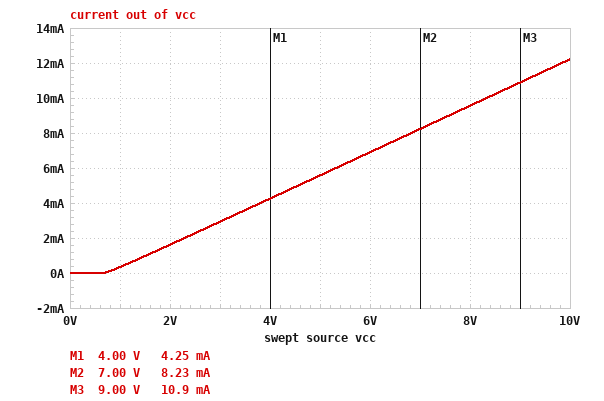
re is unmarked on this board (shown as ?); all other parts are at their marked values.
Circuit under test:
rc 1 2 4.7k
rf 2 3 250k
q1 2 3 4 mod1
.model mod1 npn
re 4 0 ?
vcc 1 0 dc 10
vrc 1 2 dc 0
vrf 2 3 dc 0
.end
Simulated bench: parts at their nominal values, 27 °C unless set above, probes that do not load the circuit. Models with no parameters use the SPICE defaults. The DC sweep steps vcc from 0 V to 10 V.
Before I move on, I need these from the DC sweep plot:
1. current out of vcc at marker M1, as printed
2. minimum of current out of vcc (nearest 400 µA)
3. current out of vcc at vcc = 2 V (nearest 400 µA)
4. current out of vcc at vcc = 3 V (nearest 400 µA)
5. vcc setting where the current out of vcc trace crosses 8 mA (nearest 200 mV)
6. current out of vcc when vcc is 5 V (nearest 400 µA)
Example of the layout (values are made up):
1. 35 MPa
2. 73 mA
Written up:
1. 4.25 mA
2. 0 A
3. 1.6 mA
4. 2.8 mA
5. 6.8 V
6. 5.6 mA
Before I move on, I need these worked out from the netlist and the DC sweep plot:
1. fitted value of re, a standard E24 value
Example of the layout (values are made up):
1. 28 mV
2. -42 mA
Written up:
1. 750 Ω
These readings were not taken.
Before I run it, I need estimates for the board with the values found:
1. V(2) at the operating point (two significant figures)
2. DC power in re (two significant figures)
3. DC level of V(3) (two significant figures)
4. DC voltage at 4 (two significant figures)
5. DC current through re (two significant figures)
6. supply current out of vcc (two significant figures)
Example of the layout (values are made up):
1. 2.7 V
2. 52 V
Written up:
1. 10 V
2. 110 mW
3. 10 V
4. 9.2 V
5. 12 mA
6. 12 mA
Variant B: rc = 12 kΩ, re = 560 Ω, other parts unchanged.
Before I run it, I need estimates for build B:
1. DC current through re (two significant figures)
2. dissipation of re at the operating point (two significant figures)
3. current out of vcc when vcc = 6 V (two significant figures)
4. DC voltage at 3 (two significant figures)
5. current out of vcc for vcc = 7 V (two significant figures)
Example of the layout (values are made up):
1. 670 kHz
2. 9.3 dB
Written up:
1. 16 mA
2. 150 mW
3. 9.2 mA
4. 10 V
5. 11 mA
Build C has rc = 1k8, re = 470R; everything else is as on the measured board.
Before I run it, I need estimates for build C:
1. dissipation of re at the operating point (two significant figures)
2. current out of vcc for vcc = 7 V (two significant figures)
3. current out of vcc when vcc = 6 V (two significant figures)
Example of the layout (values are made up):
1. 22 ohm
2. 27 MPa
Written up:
1. 180 mW
2. 13 mA
3. 11 mA
